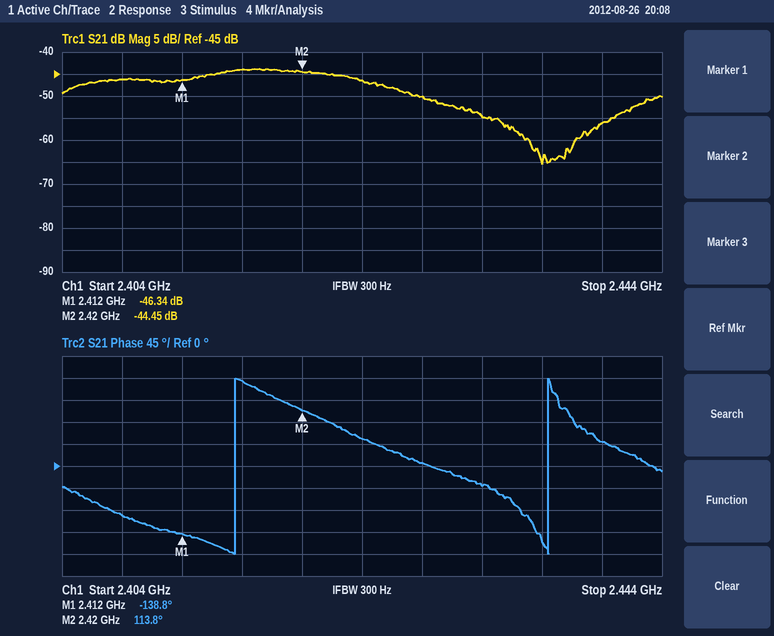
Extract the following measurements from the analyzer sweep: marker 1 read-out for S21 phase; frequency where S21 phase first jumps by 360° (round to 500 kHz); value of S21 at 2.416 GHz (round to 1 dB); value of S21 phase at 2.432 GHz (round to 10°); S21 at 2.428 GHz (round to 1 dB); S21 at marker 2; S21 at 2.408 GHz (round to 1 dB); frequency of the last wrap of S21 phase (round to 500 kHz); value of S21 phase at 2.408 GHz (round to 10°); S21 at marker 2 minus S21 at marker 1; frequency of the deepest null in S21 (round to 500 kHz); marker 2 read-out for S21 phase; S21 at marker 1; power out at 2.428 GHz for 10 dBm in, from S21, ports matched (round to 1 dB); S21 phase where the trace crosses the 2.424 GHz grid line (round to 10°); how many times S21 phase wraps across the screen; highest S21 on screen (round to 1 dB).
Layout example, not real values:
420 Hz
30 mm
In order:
-138.8°
2.4155 GHz
-44 dB
-40°
-50 dB
-44.45 dB
-46 dB
2.4365 GHz
-100°
1.89 dB
2.4360 GHz
113.8°
-46.34 dB
-40 dBm
60°
2
-44 dB
